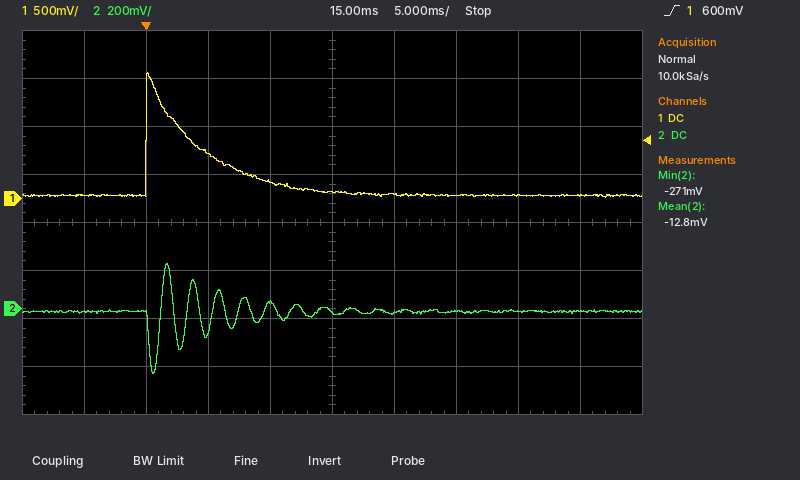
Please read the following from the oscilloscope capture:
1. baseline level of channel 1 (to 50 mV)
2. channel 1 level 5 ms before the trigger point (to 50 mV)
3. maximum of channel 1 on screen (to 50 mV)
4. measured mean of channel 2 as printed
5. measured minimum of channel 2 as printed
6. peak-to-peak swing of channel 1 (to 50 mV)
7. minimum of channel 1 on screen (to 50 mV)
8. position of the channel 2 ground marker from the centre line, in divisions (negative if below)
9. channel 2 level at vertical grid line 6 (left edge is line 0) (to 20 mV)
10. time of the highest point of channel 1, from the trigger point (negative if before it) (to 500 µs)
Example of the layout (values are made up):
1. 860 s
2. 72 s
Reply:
1. 50 mV
2. 50 mV
3. 1.30 V
4. -12.8 mV
5. -271 mV
6. 1.30 V
7. 0 mV
8. -1.8 div
9. -20 mV
10. 0.0 ms
